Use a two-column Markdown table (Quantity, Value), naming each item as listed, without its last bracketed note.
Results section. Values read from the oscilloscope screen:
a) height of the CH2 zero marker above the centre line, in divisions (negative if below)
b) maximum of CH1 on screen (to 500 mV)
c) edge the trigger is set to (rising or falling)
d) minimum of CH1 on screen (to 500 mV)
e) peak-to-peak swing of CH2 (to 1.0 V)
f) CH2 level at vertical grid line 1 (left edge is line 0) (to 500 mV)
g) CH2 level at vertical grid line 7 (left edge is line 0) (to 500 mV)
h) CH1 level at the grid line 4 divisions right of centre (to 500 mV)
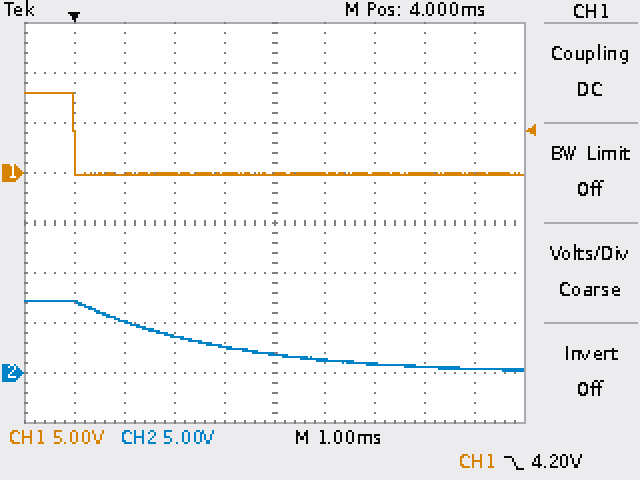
| Quantity | Value |
|---|---|
| height of the CH2 zero marker above the centre line, in divisions | -3.0 div |
| maximum of CH1 on screen | 8.0 V |
| edge the trigger is set to | falling |
| minimum of CH1 on screen | 0.0 V |
| peak-to-peak swing of CH2 | 7.0 V |
| CH2 level at vertical grid line 1 (left edge is line 0) | 7.0 V |
| CH2 level at vertical grid line 7 (left edge is line 0) | 1.0 V |
| CH1 level at the grid line 4 divisions right of centre | 0.0 V |
